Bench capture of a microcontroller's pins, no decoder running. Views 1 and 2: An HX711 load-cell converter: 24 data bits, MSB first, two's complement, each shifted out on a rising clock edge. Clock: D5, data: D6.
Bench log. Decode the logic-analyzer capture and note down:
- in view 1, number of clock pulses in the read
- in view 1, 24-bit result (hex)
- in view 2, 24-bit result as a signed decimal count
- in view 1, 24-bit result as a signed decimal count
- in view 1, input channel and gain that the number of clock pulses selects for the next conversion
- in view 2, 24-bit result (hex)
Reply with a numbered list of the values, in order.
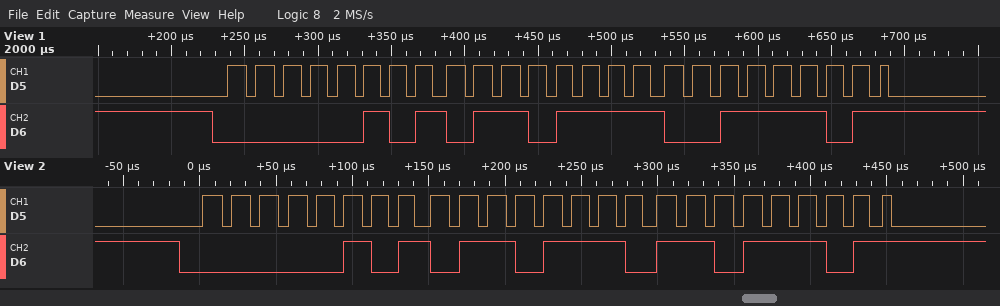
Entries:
1. 25
2. 0x056F3D
3. 356061
4. 356157
5. channel A, gain 128
6. 0x056EDD
